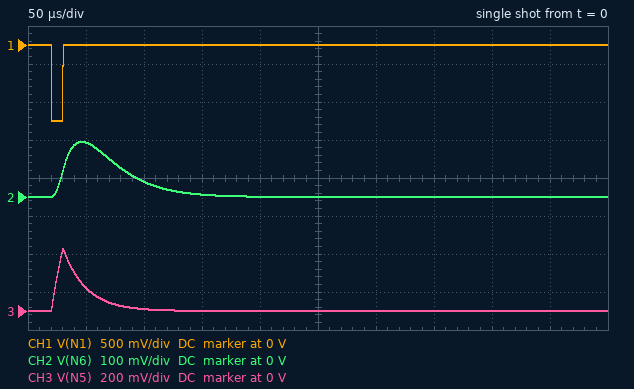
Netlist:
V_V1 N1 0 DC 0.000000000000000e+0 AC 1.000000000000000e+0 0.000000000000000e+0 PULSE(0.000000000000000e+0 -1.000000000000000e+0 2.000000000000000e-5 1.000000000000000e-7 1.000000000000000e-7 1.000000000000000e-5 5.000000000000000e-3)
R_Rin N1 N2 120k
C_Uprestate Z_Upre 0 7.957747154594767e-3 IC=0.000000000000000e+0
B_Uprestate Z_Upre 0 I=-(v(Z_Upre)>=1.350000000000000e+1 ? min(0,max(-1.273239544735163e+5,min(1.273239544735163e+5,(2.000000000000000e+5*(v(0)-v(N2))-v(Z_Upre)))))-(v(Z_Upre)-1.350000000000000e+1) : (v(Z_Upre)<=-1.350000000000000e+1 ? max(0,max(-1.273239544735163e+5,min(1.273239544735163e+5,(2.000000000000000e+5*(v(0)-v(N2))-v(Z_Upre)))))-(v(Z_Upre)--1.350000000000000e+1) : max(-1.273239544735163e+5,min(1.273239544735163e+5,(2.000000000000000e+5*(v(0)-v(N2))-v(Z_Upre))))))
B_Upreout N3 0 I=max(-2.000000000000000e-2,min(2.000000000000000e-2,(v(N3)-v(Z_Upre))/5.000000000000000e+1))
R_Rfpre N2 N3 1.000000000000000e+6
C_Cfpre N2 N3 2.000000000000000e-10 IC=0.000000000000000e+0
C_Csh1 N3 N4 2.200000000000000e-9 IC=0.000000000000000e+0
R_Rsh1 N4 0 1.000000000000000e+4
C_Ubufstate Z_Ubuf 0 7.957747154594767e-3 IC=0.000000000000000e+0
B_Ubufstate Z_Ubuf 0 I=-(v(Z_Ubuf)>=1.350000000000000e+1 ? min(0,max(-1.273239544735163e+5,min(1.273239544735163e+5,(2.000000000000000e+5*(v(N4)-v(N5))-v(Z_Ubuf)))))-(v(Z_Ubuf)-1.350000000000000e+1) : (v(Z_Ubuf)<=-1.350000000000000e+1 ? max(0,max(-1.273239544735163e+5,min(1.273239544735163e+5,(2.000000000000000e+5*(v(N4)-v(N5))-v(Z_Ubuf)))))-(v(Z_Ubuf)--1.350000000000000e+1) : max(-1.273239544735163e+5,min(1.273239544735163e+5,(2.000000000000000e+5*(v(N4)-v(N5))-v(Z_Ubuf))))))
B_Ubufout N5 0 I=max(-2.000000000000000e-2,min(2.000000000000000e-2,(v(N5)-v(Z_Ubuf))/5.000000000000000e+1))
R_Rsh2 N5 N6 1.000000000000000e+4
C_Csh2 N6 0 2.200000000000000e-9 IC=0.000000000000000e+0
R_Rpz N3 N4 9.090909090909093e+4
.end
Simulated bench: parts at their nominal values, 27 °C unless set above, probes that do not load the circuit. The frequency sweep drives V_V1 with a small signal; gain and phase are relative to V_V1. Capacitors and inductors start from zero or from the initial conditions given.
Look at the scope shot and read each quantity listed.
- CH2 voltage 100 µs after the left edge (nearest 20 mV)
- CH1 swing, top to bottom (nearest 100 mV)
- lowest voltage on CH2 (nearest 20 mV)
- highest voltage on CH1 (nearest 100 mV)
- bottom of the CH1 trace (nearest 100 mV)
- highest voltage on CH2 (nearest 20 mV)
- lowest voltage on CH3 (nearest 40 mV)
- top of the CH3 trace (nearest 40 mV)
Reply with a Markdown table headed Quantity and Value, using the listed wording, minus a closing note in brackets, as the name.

| Quantity | Value |
|---|---|
| CH2 voltage 100 µs after the left edge | 40 mV |
| CH1 swing, top to bottom | 1.0 V |
| lowest voltage on CH2 | 0 V |
| highest voltage on CH1 | 0 V |
| bottom of the CH1 trace | -1.0 V |
| highest voltage on CH2 | 140 mV |
| lowest voltage on CH3 | 0 V |
| top of the CH3 trace | 320 mV |
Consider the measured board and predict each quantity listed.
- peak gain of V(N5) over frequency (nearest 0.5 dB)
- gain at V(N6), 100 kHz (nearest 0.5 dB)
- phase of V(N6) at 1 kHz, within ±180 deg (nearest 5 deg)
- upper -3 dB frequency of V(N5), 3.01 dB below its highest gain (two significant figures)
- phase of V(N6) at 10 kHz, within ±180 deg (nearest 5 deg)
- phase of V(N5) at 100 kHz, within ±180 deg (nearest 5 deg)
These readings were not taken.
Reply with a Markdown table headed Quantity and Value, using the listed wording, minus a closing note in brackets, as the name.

| Quantity | Value |
|---|---|
| peak gain of V(N5) over frequency | -1.5 dB |
| gain at V(N6), 100 kHz | -46.5 dB |
| phase of V(N6) at 1 kHz, within ±180 deg | 165 deg |
| upper -3 dB frequency of V(N5), 3.01 dB below its highest gain | 8.0 kHz |
| phase of V(N6) at 10 kHz, within ±180 deg | 75 deg |
| phase of V(N5) at 100 kHz, within ±180 deg | 90 deg |
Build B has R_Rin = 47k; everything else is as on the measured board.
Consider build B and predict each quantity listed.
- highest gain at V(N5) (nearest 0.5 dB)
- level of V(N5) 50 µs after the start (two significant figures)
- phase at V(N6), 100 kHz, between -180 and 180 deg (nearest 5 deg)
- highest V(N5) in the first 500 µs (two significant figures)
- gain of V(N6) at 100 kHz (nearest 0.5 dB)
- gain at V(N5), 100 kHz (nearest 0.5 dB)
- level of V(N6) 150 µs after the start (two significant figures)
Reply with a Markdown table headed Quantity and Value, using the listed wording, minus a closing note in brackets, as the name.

| Quantity | Value |
|---|---|
| highest gain at V(N5) | 6.5 dB |
| level of V(N5) 50 µs after the start | 310 mV |
| phase at V(N6), 100 kHz, between -180 and 180 deg | 5 deg |
| highest V(N5) in the first 500 µs | 840 mV |
| gain of V(N6) at 100 kHz | -38.5 dB |
| gain at V(N5), 100 kHz | -15.5 dB |
| level of V(N6) 150 µs after the start | 16 mV |
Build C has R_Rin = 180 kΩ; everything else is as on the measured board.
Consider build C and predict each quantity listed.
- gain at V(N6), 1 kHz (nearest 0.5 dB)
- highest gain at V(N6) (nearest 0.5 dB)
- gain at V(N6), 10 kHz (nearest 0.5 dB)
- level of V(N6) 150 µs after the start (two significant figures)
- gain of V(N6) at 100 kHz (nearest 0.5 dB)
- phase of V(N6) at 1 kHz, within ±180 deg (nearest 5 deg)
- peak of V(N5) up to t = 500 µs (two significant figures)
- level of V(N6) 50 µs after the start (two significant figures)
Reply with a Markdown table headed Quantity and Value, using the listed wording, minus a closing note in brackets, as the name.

| Quantity | Value |
|---|---|
| gain at V(N6), 1 kHz | -5.5 dB |
| highest gain at V(N6) | -5.0 dB |
| gain at V(N6), 10 kHz | -14.0 dB |
| level of V(N6) 150 µs after the start | 4.1 mV |
| gain of V(N6) at 100 kHz | -50.0 dB |
| phase of V(N6) at 1 kHz, within ±180 deg | 165 deg |
| peak of V(N5) up to t = 500 µs | 220 mV |
| level of V(N6) 50 µs after the start | 96 mV |
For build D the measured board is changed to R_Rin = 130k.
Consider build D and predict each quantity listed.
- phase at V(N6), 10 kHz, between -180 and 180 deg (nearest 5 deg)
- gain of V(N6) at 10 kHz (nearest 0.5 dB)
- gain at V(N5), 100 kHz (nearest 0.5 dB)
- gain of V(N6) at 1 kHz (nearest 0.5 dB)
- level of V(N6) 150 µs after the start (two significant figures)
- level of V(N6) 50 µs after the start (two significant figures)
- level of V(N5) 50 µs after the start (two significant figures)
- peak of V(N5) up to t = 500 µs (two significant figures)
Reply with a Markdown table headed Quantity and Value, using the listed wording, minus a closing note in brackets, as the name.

| Quantity | Value |
|---|---|
| phase at V(N6), 10 kHz, between -180 and 180 deg | 75 deg |
| gain of V(N6) at 10 kHz | -11.0 dB |
| gain at V(N5), 100 kHz | -24.5 dB |
| gain of V(N6) at 1 kHz | -2.5 dB |
| level of V(N6) 150 µs after the start | 5.7 mV |
| level of V(N6) 50 µs after the start | 130 mV |
| level of V(N5) 50 µs after the start | 110 mV |
| peak of V(N5) up to t = 500 µs | 300 mV |
